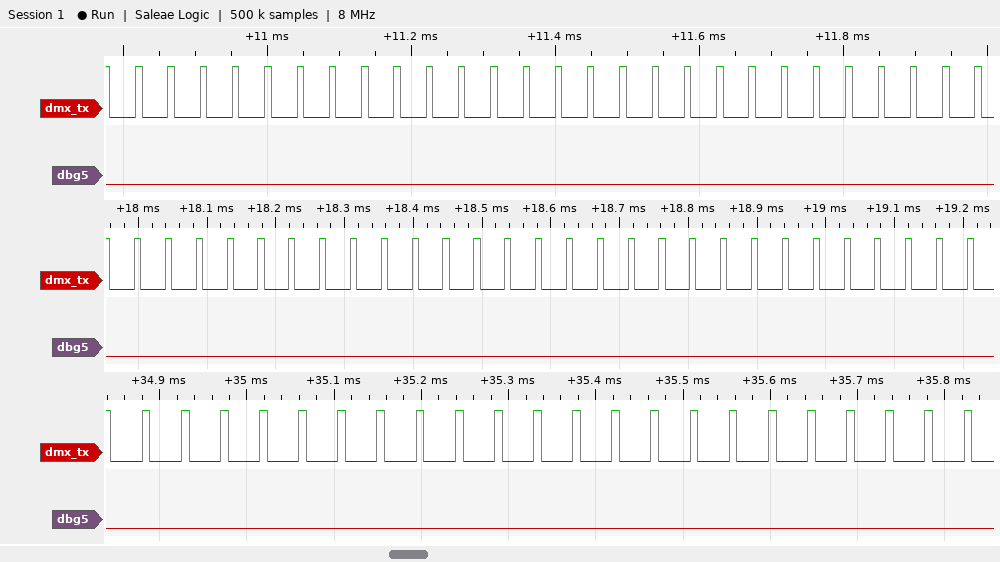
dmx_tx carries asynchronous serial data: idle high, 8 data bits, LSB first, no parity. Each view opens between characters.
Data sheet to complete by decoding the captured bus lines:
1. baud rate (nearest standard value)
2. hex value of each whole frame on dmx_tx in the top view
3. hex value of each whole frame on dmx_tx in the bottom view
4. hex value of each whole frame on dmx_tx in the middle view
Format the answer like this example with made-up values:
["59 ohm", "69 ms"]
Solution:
["115200 baud", "08, 08, 08, 08, 08, 08, 08, 08, 08, 08, 08, 08, 08", "08, 08, 08, 08, 08, 08, 08, 08, 08, 08, 08", "08, 08, 08, 08, 08, 08, 08, 08, 08, 08, 08, 08, 08, 08"]
